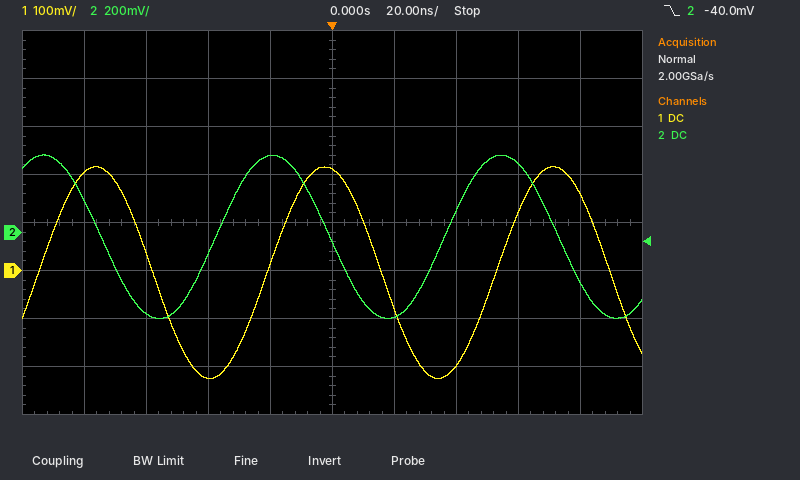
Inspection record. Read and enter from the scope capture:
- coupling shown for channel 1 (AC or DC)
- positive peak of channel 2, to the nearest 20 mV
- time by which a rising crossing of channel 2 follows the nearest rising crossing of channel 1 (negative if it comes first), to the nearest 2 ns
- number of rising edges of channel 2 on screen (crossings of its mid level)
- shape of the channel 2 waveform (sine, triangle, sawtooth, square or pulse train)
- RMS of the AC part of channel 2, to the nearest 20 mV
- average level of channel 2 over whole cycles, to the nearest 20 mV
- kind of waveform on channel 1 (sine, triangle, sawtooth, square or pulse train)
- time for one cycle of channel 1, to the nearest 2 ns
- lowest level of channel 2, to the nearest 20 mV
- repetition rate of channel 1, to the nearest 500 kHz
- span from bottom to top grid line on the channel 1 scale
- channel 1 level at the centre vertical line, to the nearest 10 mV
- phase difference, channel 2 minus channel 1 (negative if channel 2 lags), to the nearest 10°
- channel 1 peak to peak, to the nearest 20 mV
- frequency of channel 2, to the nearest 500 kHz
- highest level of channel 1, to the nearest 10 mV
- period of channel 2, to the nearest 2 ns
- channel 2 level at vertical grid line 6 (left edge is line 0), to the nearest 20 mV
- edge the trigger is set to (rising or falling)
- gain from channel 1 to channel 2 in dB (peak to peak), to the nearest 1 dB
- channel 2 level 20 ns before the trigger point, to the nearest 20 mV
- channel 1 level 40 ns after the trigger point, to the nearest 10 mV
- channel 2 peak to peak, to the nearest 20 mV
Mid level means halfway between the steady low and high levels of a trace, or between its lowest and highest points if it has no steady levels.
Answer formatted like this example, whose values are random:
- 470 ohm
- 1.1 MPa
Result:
- DC
- 320 mV
- -16 ns
- 2
- sine
- 240 mV
- -20 mV
- sine
- 74 ns
- -360 mV
- 13.5 MHz
- 800 mV
- 210 mV
- +80°
- 440 mV
- 13.5 MHz
- 220 mV
- 74 ns
- -360 mV
- falling
- 4 dB
- 320 mV
- -200 mV
- 680 mV
